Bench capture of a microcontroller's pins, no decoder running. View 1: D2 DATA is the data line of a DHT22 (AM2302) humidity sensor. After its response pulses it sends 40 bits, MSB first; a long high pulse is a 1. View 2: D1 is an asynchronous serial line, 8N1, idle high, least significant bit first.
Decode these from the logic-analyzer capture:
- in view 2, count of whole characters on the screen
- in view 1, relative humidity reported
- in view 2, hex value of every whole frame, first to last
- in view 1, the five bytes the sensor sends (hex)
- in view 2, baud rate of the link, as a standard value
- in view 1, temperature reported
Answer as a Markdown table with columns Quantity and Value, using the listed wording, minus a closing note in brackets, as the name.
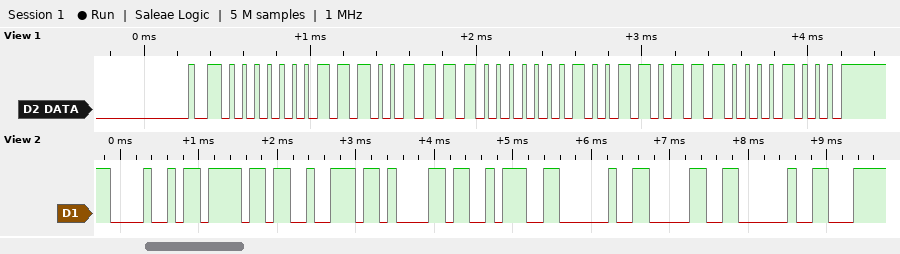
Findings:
| Quantity | Value |
|---|---|
| in view 2, count of whole characters on the screen | 8 |
| in view 1, relative humidity reported | 46.3 % |
| in view 2, hex value of every whole frame, first to last | 0x48 0x6F 0x72 0x61 0x3A 0x20 0x30 0x20 |
| in view 1, the five bytes the sensor sends | 01 CF 01 37 08 |
| in view 2, baud rate of the link, as a standard value | 9600 baud |
| in view 1, temperature reported | 31.1 °C |
